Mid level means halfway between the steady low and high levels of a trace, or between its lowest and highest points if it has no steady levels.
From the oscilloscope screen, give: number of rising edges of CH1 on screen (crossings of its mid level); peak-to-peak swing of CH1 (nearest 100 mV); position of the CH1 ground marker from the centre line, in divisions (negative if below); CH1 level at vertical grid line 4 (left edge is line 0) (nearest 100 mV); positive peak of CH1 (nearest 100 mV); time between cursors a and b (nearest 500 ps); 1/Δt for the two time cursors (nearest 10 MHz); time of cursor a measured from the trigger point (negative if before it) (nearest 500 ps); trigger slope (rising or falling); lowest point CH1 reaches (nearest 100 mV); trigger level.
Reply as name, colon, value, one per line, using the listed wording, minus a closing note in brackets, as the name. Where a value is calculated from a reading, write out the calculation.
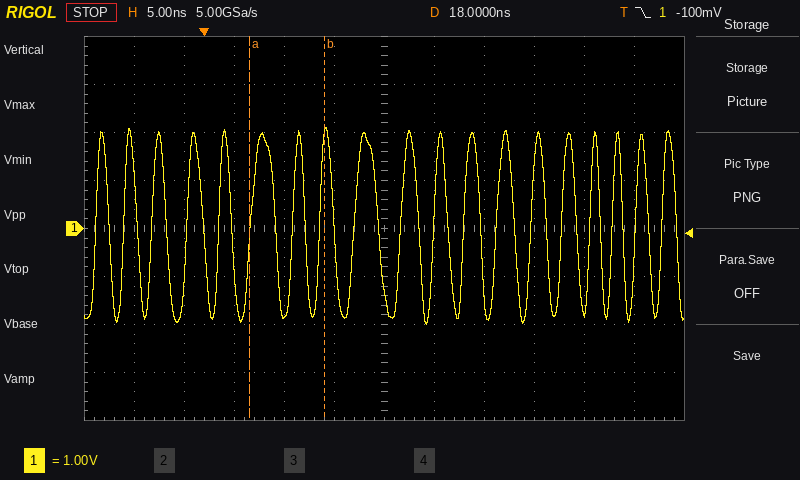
number of rising edges of CH1 on screen: 19
peak-to-peak swing of CH1: 2.1 V − (-2.0 V) = 4.1 V
position of the CH1 ground marker from the centre line, in divisions: 0.0 div
CH1 level at vertical grid line 4 (left edge is line 0): -1.8 V
positive peak of CH1: 2.1 V
time between cursors a and b: 7.5 ns
1/Δt for the two time cursors: 1 / 7.5 ns ≈ 130 MHz
time of cursor a measured from the trigger point (negative if before it): +4.5 ns
trigger slope: falling
lowest point CH1 reaches: -2.0 V
trigger level: -100 mV
